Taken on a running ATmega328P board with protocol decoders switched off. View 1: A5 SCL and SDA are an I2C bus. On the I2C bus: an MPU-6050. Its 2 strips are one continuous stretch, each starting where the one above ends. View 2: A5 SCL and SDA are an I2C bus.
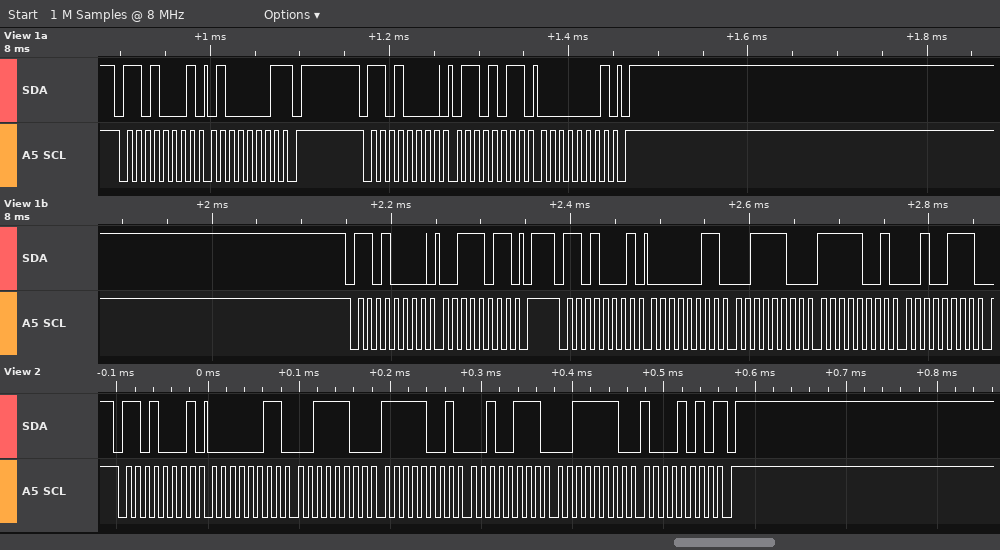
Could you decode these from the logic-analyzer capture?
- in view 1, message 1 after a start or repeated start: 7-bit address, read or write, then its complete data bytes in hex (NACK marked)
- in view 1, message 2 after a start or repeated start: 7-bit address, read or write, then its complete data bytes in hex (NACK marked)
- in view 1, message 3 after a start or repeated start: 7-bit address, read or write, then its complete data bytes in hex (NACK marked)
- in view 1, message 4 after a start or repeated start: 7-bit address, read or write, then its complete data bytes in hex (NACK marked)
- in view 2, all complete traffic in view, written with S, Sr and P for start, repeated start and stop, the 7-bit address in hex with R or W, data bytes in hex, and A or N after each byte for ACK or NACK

0x68 read: 41 NACK
0x68 write: 6B 01
0x68 write: 3B
0x68 read: 03 3C F9 27
S 68R A 03 A 3C A F9 A 27 A 3E A 8A N P
